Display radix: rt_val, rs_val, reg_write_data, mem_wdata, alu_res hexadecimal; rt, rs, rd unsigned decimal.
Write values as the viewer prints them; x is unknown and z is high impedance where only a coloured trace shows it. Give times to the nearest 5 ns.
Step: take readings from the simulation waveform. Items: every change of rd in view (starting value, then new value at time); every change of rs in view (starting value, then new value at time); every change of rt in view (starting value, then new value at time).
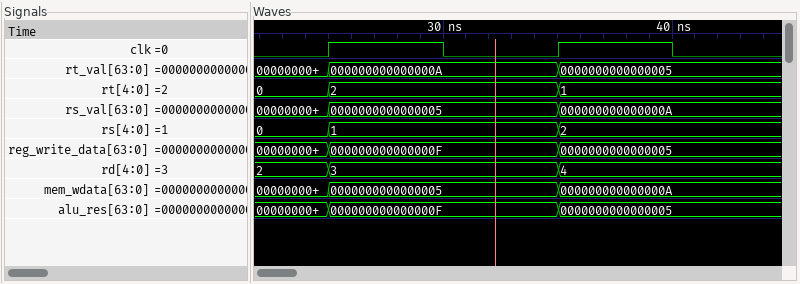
2, 3 at 25 ns, 4 at 35 ns
0, 1 at 25 ns, 2 at 35 ns
0, 2 at 25 ns, 1 at 35 ns
